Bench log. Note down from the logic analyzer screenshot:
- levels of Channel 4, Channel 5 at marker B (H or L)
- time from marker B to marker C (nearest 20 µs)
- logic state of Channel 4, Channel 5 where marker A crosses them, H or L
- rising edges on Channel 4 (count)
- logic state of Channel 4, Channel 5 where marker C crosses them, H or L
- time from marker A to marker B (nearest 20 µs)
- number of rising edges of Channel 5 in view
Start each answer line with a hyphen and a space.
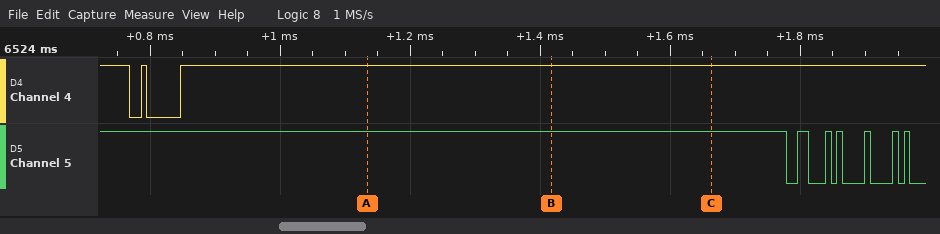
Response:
- Channel 4=H, Channel 5=H
- 240 µs
- Channel 4=H, Channel 5=H
- 2
- Channel 4=H, Channel 5=H
- 280 µs
- 6
